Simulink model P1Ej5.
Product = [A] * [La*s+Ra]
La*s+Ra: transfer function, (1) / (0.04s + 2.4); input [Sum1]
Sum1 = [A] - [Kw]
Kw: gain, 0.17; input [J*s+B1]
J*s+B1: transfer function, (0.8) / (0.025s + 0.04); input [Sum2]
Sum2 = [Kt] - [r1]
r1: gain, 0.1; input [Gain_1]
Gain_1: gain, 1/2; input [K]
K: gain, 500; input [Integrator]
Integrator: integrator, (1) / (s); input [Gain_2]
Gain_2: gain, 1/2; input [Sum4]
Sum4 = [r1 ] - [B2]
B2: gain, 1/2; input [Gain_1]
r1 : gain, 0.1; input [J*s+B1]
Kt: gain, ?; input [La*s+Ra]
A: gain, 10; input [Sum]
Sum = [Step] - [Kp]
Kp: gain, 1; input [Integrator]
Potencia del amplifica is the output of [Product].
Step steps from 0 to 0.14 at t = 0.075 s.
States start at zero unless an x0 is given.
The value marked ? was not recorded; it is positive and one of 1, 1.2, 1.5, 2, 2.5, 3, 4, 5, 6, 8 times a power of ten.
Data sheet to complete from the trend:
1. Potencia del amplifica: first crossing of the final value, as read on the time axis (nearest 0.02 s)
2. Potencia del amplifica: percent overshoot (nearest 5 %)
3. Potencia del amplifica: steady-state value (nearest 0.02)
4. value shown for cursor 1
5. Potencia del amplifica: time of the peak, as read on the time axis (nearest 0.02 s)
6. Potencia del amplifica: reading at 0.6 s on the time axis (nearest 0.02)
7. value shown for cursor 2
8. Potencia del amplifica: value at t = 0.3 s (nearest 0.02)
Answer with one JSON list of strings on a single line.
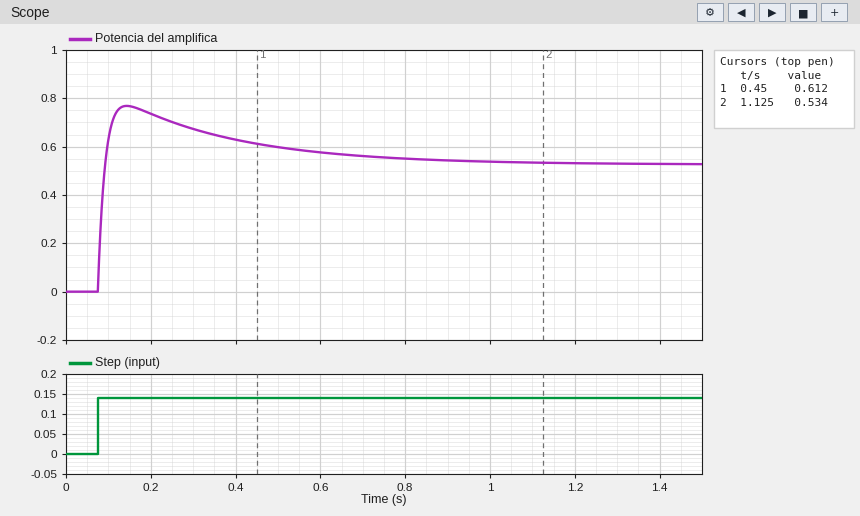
["0.10 s", "45 %", "0.52", "0.612", "0.14 s", "0.58", "0.534", "0.68"]
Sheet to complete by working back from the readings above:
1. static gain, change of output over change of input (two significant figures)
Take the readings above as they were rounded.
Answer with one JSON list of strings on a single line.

["3.7"]
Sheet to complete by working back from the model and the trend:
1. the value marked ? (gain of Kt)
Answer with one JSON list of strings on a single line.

["0.5"]
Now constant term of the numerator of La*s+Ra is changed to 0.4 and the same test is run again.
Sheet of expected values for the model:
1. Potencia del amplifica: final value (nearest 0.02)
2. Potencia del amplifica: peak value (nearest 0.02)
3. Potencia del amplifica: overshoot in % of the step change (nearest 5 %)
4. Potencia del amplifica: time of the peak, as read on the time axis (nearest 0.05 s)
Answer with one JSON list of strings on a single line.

["0.26", "0.32", "20 %", "0.15 s"]
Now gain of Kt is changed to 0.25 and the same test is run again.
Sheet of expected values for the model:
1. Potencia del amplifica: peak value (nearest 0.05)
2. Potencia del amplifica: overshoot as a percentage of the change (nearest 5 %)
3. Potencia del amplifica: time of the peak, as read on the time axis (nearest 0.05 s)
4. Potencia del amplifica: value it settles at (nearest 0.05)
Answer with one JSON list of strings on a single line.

["0.80", "25 %", "0.15 s", "0.65"]
